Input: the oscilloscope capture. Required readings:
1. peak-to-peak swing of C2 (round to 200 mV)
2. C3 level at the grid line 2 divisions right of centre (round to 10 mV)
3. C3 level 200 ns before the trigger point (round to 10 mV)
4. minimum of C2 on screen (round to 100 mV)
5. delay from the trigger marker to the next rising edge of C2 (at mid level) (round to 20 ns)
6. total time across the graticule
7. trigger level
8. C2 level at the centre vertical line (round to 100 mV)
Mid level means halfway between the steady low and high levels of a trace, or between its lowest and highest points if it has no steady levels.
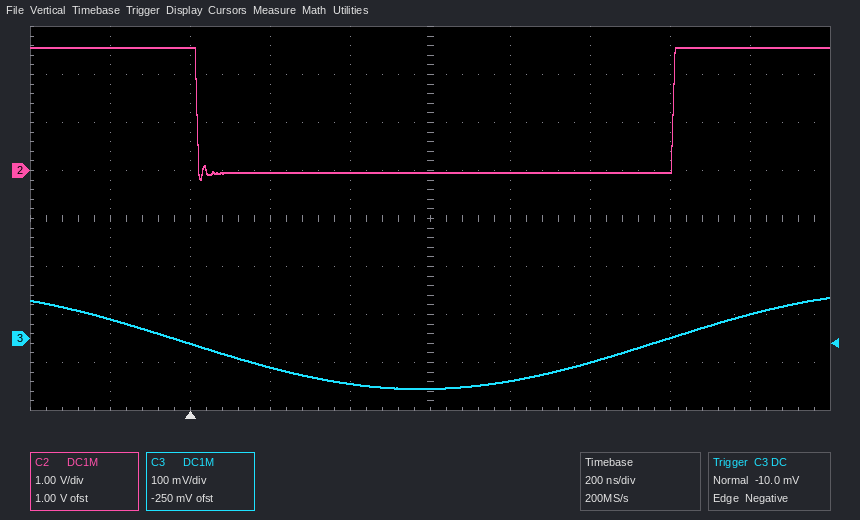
2.8 V
-50 mV
40 mV
-200 mV
1.20 µs
2 µs
-10.0 mV
0.0 V
